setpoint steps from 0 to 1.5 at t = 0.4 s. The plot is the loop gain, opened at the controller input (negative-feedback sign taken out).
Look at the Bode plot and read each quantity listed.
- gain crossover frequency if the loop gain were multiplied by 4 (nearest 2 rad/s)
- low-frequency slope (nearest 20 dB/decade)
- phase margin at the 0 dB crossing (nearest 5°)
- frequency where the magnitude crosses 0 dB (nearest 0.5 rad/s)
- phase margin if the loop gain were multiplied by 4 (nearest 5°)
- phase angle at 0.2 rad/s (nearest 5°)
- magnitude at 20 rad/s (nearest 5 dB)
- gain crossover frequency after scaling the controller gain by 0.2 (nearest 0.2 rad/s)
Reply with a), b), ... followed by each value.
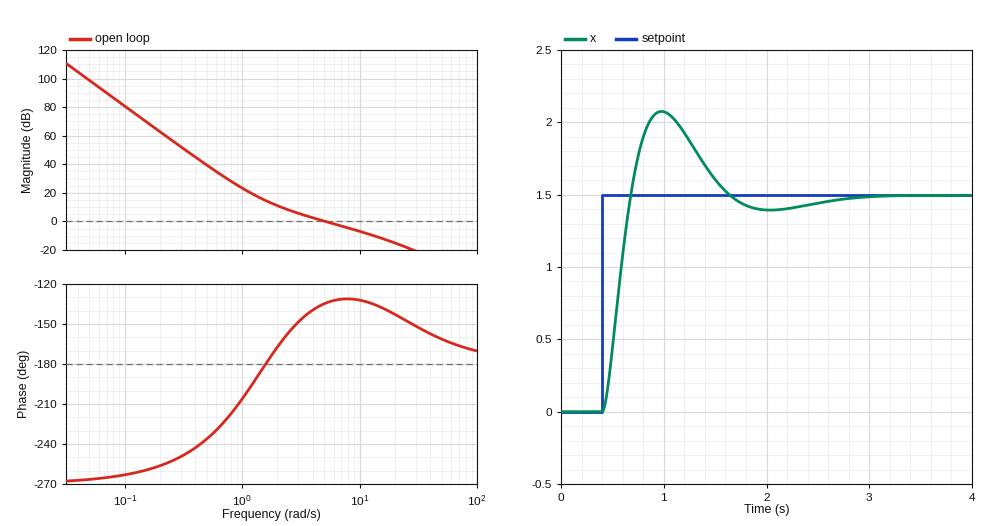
a) 16 rad/s
b) -60 dB/decade
c) 45°
d) 5.0 rad/s
e) 40°
f) -255°
g) -15 dB
h) 1.6 rad/s
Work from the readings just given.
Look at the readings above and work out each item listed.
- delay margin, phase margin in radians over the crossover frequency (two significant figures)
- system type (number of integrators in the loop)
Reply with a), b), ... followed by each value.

a) 0.16 s
b) 3
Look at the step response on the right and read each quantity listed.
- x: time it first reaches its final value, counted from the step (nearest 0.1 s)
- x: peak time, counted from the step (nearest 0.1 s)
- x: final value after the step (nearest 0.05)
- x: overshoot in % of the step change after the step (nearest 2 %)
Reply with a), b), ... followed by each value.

a) 0.3 s
b) 0.6 s
c) 1.50
d) 38 %
